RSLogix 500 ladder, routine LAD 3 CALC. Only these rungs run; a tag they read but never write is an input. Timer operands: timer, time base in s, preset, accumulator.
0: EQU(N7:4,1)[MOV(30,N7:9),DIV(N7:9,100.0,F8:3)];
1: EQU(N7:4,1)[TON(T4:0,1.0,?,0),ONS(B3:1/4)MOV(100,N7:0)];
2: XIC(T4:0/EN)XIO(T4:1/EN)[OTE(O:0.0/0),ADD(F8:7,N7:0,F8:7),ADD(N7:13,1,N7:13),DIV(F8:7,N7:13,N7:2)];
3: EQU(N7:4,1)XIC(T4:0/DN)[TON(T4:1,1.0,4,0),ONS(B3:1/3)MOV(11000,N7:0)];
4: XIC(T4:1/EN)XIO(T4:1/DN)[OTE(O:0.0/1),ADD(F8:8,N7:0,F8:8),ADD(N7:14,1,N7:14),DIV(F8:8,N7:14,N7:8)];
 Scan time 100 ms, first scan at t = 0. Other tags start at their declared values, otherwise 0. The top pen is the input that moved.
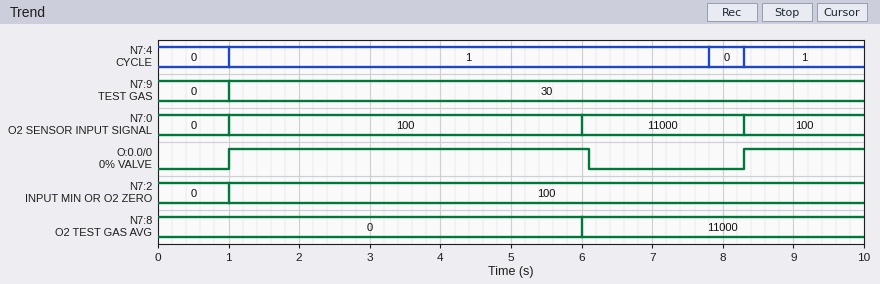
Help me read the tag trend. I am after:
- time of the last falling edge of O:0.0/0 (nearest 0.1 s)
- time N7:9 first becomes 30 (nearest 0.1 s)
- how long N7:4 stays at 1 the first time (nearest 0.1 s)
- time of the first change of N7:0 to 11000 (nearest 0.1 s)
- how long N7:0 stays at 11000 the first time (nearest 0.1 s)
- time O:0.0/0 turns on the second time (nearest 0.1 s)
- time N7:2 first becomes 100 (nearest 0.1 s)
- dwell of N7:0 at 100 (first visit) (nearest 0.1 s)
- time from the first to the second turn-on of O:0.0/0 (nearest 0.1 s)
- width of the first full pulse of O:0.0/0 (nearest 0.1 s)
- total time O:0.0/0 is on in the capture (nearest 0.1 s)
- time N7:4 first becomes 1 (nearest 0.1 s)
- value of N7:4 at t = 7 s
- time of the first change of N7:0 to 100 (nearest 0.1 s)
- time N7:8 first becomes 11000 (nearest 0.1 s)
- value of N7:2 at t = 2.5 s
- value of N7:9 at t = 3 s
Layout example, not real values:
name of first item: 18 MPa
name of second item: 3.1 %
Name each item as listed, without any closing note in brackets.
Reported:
time of the last falling edge of O:0.0/0: 6.1 s
time N7:9 first becomes 30: 1.0 s
how long N7:4 stays at 1 the first time: 6.8 s
time of the first change of N7:0 to 11000: 6.0 s
how long N7:0 stays at 11000 the first time: 2.3 s
time O:0.0/0 turns on the second time: 8.3 s
time N7:2 first becomes 100: 1.0 s
dwell of N7:0 at 100 (first visit): 5.0 s
time from the first to the second turn-on of O:0.0/0: 7.3 s
width of the first full pulse of O:0.0/0: 5.1 s
total time O:0.0/0 is on in the capture: 6.8 s
time N7:4 first becomes 1: 1.0 s
value of N7:4 at t = 7 s: 1
time of the first change of N7:0 to 100: 1.0 s
time N7:8 first becomes 11000: 6.0 s
value of N7:2 at t = 2.5 s: 100
value of N7:9 at t = 3 s: 30
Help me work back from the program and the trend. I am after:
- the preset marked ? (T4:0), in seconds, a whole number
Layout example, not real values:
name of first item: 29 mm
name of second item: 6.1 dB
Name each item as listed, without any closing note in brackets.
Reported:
the preset marked ? (T4:0), in seconds, a whole number: 5 s
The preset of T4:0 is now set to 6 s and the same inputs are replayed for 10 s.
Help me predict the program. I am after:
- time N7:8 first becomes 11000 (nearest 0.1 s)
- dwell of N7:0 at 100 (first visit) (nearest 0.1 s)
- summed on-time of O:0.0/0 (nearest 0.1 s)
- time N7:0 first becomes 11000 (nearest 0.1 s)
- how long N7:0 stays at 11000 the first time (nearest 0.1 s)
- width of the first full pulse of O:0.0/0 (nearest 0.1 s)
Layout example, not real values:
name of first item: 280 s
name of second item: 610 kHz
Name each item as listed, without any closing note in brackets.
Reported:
time N7:8 first becomes 11000: 7.0 s
dwell of N7:0 at 100 (first visit): 6.0 s
summed on-time of O:0.0/0: 7.8 s
time N7:0 first becomes 11000: 7.0 s
how long N7:0 stays at 11000 the first time: 1.3 s
width of the first full pulse of O:0.0/0: 6.1 s
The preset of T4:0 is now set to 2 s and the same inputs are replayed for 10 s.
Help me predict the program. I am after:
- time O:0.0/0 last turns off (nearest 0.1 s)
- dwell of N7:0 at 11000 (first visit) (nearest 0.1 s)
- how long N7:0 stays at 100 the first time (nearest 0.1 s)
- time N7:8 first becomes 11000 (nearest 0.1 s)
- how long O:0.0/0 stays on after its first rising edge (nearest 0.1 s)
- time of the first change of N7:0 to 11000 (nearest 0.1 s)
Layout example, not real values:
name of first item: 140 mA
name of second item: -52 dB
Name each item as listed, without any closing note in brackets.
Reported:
time O:0.0/0 last turns off: 3.1 s
dwell of N7:0 at 11000 (first visit): 5.3 s
how long N7:0 stays at 100 the first time: 2.0 s
time N7:8 first becomes 11000: 3.0 s
how long O:0.0/0 stays on after its first rising edge: 2.1 s
time of the first change of N7:0 to 11000: 3.0 s
